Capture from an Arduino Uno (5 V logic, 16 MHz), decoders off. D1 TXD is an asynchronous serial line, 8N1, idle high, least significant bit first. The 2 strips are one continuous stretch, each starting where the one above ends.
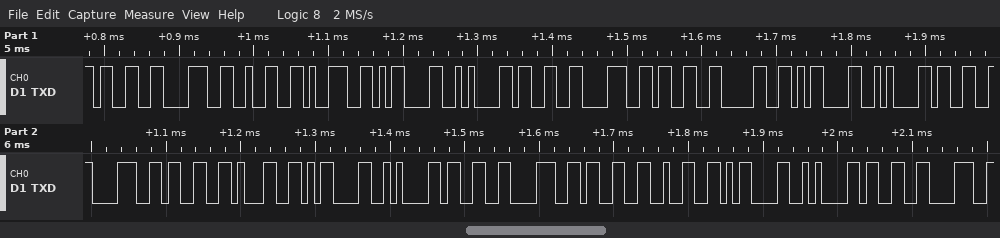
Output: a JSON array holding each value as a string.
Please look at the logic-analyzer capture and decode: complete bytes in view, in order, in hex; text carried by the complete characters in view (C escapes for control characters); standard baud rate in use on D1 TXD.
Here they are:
["33 38 32 39 0D 0A 33 38 33 30 0D 0A 33 38 33 31 0D 0A 33 38 33 32 0D 0A 33 38", "\"3829\\r\\n3830\\r\\n3831\\r\\n3832\\r\\n38\"", "115200 baud"]
